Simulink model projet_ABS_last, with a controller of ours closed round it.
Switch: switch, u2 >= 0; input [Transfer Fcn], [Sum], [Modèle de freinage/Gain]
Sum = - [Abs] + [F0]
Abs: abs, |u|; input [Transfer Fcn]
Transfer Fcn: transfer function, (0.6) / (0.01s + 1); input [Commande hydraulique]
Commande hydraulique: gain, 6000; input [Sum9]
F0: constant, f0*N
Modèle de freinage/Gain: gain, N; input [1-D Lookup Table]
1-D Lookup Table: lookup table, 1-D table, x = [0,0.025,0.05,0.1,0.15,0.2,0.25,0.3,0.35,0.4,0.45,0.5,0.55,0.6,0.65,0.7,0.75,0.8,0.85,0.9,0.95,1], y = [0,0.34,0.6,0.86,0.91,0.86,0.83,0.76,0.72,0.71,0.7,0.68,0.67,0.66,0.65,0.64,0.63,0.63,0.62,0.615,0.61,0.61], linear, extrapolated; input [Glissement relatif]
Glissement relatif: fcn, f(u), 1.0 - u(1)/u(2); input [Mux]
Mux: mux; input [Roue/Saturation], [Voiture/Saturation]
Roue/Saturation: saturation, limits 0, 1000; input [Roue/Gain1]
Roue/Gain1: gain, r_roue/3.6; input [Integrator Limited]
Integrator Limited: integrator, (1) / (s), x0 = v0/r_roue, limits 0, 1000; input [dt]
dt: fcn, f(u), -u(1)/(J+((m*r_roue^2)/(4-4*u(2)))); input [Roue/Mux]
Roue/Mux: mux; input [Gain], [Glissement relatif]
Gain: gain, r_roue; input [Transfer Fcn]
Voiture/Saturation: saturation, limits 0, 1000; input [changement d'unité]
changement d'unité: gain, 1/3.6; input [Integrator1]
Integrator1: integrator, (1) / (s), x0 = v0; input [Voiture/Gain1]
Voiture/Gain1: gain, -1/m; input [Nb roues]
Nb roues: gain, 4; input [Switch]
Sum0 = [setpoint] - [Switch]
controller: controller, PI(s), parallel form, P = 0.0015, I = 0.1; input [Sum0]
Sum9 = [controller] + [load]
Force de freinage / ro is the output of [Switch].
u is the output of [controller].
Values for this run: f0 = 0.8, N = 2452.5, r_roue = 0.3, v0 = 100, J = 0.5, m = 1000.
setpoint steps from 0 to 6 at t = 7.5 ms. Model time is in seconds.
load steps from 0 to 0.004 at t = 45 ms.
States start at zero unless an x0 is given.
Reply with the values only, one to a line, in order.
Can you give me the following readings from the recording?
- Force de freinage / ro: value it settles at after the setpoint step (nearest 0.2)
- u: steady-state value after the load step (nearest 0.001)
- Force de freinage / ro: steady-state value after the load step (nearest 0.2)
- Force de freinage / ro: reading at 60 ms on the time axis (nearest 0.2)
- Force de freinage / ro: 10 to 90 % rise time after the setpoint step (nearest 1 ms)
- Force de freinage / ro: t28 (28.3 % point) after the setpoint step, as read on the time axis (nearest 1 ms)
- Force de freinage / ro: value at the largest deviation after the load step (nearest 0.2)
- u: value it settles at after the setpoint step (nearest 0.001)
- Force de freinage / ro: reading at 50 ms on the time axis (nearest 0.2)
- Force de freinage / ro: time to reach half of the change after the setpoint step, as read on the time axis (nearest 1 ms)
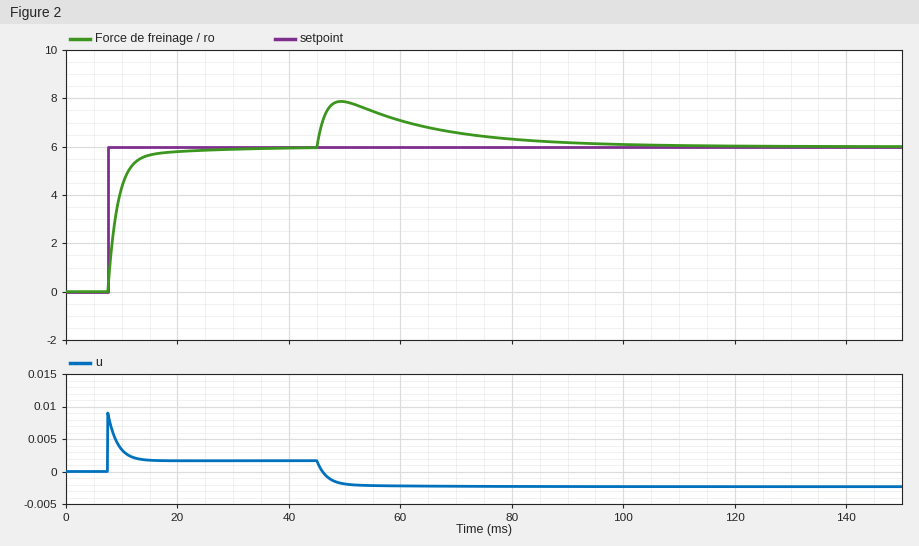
6.0
-0.002
6.0
7.0
5 ms
8 ms
7.8
0.002
7.8
9 ms
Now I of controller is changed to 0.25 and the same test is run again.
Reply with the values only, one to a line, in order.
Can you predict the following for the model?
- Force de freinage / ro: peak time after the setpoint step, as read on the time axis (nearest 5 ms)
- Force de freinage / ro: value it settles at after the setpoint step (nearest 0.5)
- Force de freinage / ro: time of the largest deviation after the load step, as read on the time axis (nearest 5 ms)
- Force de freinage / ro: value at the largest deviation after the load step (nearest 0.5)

15 ms
6.0
50 ms
7.5
